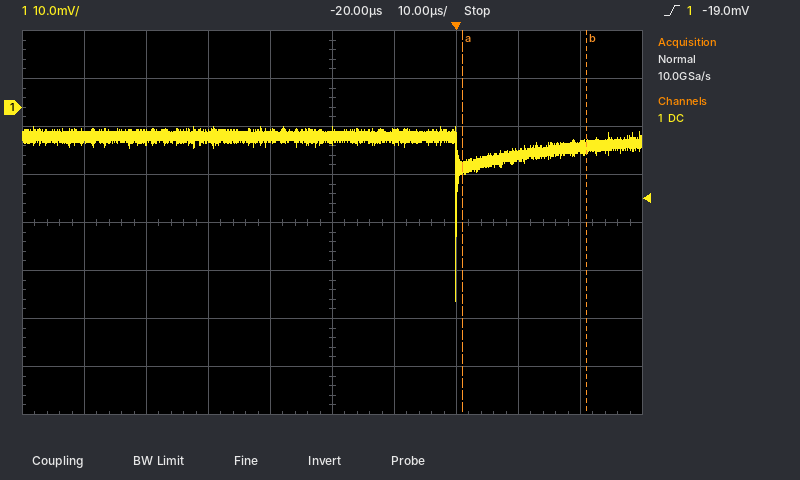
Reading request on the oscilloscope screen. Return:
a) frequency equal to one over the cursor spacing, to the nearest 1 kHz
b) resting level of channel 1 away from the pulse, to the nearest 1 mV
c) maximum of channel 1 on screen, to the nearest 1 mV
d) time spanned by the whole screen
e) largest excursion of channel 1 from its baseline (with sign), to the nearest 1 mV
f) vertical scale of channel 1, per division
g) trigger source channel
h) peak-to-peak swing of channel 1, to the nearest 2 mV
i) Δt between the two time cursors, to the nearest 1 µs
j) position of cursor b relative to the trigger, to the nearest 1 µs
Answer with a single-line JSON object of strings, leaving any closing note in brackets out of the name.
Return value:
{"frequency equal to one over the cursor spacing, to the nearest 1 kHz": "50 kHz", "resting level of channel 1 away from the pulse, to the nearest 1 mV": "-6 mV", "maximum of channel 1 on screen, to the nearest 1 mV": "-4 mV", "time spanned by the whole screen": "100 µs", "largest excursion of channel 1 from its baseline (with sign), to the nearest 1 mV": "-34 mV", "vertical scale of channel 1, per division": "10 mV", "trigger source channel": "channel 1", "peak-to-peak swing of channel 1, to the nearest 2 mV": "36 mV", "Δt between the two time cursors, to the nearest 1 µs": "20 µs", "position of cursor b relative to the trigger, to the nearest 1 µs": "+21 µs"}
